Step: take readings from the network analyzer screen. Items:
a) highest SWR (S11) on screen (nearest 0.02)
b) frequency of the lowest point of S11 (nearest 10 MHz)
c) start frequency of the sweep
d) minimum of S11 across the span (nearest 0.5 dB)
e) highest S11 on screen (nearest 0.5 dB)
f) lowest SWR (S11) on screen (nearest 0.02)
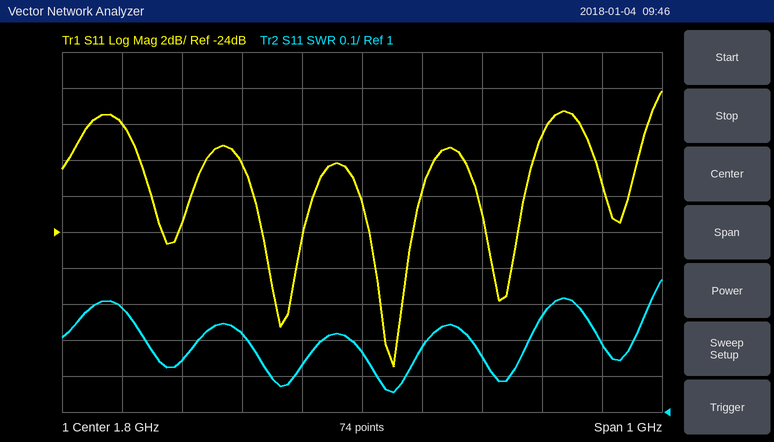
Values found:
1.36
1.85 GHz
1.3 GHz
-31.5 dB
-16.0 dB
1.06
